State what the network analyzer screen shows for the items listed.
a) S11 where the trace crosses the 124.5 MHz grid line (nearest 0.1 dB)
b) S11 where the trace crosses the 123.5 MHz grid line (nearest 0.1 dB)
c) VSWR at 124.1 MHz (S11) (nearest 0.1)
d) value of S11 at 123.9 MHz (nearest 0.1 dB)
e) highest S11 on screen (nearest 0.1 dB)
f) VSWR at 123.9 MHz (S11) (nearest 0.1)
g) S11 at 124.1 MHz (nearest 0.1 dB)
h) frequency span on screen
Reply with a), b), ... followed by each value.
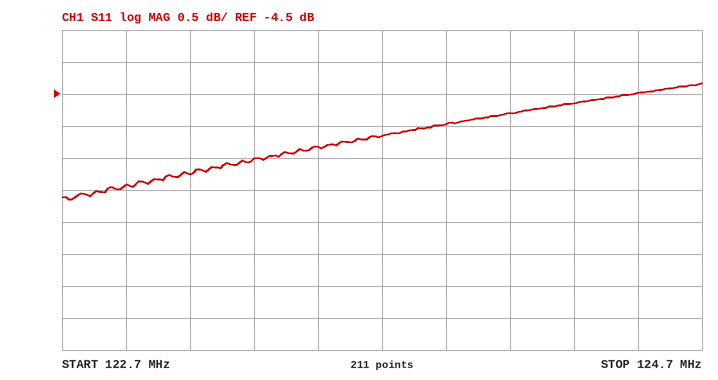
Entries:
a) -4.5 dB
b) -5.3 dB
c) 3.7
d) -5.0 dB
e) -4.3 dB
f) 3.6
g) -4.8 dB
h) 2 MHz
